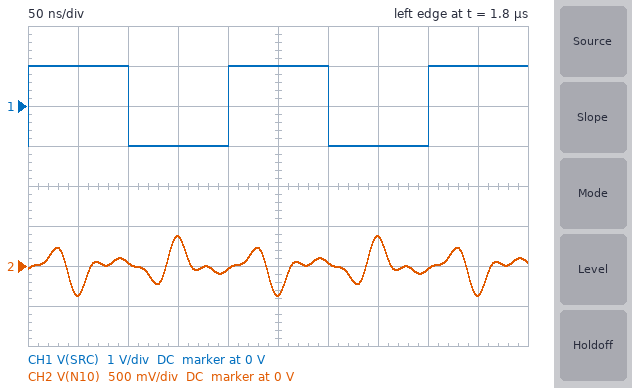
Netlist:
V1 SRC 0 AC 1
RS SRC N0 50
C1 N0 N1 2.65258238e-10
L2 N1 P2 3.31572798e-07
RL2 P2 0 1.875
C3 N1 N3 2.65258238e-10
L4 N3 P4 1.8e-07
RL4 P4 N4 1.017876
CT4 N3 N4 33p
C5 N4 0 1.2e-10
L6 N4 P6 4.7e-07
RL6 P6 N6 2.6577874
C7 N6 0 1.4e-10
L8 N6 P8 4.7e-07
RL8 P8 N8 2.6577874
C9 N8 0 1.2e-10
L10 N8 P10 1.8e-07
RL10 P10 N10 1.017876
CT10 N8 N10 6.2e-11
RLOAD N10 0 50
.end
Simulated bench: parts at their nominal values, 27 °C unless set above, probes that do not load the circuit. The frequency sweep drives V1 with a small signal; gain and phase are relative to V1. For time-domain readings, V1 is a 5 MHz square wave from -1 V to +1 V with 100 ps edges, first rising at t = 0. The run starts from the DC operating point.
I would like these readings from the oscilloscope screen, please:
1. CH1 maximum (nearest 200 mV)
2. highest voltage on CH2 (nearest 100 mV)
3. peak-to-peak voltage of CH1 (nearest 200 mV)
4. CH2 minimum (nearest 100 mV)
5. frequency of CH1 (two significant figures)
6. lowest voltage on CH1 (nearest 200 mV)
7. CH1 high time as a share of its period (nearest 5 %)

1.0 V
400 mV
2.0 V
-400 mV
5.0 MHz
-1.0 V
50 %
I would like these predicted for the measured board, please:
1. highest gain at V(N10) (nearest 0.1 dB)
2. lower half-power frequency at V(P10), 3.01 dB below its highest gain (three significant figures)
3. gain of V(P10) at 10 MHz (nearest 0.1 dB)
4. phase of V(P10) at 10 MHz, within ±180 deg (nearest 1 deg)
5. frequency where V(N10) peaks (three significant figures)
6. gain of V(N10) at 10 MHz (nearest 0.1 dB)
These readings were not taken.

-7.2 dB
12.9 MHz
-13.5 dB
67 deg
21.6 MHz
-13.7 dB
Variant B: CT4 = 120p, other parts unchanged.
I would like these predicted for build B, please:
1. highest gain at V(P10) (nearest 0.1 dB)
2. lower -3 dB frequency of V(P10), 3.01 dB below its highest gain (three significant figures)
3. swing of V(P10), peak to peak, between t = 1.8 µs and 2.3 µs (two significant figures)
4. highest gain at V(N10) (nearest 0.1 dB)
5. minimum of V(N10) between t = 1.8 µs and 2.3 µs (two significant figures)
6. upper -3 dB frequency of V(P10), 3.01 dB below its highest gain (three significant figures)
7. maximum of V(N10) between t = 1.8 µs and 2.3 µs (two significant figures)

-7.2 dB
12.5 MHz
610 mV
-7.4 dB
-300 mV
29.7 MHz
300 mV
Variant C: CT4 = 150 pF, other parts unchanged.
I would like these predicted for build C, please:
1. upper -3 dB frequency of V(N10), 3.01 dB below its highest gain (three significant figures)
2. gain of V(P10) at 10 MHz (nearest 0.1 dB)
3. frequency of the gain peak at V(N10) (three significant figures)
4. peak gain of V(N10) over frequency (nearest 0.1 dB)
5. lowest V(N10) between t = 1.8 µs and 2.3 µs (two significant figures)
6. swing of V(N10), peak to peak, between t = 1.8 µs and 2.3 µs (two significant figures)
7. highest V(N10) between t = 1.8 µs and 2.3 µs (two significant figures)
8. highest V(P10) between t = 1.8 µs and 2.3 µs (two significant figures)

26.9 MHz
-13.5 dB
19.0 MHz
-7.5 dB
-280 mV
560 mV
280 mV
290 mV
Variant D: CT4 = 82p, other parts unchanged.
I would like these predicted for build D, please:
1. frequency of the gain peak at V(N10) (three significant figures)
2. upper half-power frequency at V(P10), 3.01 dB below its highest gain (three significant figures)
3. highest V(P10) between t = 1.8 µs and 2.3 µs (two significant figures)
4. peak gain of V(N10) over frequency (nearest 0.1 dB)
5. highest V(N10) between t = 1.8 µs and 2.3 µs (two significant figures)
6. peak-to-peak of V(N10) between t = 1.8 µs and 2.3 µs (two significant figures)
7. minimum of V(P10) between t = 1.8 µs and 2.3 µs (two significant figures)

20.5 MHz
33.9 MHz
360 mV
-7.3 dB
350 mV
700 mV
-360 mV
